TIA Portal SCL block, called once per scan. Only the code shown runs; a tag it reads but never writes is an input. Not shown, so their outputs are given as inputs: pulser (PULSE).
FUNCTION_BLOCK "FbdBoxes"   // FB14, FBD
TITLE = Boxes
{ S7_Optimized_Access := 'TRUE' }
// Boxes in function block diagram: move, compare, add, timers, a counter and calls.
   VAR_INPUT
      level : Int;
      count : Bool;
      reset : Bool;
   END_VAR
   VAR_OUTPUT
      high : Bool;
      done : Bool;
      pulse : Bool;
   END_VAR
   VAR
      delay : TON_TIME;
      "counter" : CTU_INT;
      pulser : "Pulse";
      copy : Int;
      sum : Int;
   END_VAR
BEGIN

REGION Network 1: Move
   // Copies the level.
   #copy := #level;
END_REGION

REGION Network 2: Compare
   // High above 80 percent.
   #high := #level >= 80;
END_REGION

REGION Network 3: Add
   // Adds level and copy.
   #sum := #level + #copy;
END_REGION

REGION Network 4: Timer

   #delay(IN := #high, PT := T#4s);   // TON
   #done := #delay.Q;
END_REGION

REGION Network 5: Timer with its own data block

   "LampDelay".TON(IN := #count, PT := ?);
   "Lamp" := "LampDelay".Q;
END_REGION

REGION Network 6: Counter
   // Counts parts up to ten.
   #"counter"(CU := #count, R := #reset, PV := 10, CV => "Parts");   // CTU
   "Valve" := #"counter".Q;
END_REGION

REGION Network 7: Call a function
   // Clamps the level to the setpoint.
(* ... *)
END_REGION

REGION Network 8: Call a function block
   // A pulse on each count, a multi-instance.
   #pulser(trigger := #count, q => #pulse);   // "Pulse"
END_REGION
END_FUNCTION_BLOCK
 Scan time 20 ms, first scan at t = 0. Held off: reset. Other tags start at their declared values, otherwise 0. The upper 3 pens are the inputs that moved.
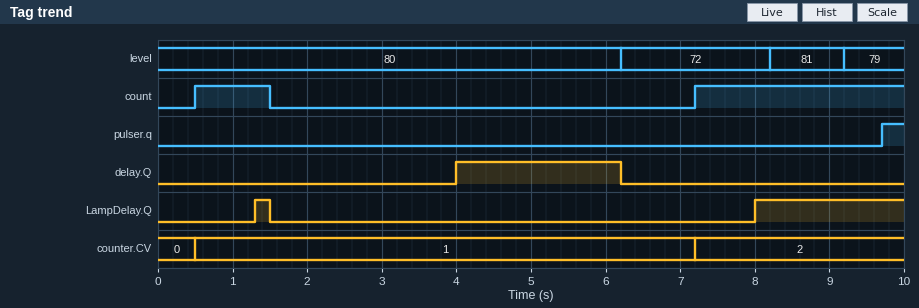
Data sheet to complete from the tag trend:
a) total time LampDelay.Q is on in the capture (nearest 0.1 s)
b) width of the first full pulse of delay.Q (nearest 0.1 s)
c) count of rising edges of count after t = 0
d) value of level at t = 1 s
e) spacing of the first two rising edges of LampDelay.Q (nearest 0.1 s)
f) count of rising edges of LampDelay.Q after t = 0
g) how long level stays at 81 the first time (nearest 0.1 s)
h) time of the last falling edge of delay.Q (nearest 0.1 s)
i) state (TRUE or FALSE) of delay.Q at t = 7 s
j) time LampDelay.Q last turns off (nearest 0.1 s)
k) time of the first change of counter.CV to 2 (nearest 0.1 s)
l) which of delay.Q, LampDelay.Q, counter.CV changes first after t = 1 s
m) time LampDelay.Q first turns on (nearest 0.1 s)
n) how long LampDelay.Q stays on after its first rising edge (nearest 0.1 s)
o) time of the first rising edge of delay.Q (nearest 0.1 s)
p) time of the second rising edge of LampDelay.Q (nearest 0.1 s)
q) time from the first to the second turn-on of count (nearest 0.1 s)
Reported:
2.2 s
2.2 s
2
80
6.7 s
2
1.0 s
6.2 s
FALSE
1.5 s
7.2 s
LampDelay.Q
1.3 s
0.2 s
4.0 s
8.0 s
6.7 s
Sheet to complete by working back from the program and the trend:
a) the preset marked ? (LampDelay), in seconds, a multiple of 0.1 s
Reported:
0.8 s
